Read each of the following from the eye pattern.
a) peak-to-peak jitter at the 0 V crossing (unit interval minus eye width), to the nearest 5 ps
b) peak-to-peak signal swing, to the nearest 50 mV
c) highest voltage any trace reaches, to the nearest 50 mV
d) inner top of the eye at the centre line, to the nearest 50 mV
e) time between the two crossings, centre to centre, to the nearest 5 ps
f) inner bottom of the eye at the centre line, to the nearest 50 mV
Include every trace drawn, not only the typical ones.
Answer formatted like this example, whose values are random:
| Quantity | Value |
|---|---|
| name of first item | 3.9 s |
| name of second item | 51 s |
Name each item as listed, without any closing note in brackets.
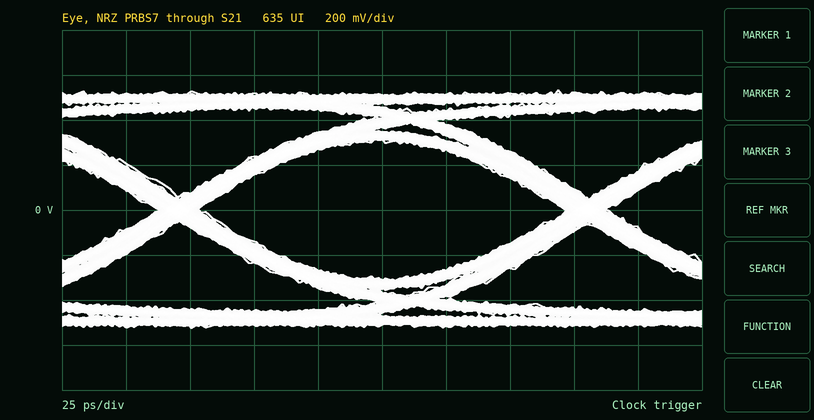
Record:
| Quantity | Value |
|---|---|
| peak-to-peak jitter at the 0 V crossing (unit interval minus eye width), to the nearest 5 ps | 15 ps |
| peak-to-peak signal swing, to the nearest 50 mV | 1.05 V |
| highest voltage any trace reaches, to the nearest 50 mV | 550 mV |
| inner top of the eye at the centre line, to the nearest 50 mV | 300 mV |
| time between the two crossings, centre to centre, to the nearest 5 ps | 160 ps |
| inner bottom of the eye at the centre line, to the nearest 50 mV | -300 mV |
